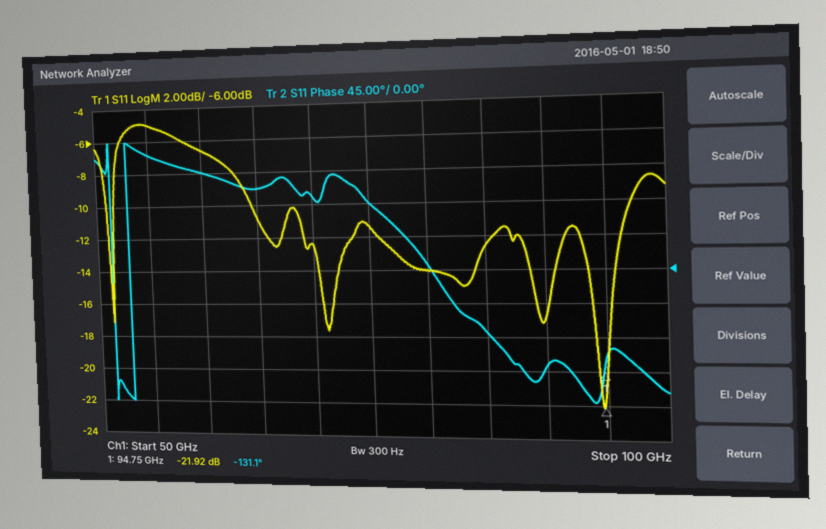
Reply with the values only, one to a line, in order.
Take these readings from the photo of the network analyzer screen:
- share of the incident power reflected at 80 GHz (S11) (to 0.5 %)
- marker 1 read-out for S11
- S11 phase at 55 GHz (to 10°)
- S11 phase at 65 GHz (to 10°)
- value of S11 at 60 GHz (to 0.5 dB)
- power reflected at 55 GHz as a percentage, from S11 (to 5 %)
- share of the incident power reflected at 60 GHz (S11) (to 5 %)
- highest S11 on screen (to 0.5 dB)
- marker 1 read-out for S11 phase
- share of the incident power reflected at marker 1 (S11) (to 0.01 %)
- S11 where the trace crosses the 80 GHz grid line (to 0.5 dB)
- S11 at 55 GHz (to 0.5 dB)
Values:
4.0 %
-21.92 dB
160°
110°
-6.5 dB
30 %
20 %
-5.0 dB
-131.1°
0.64 %
-14.0 dB
-5.0 dB
